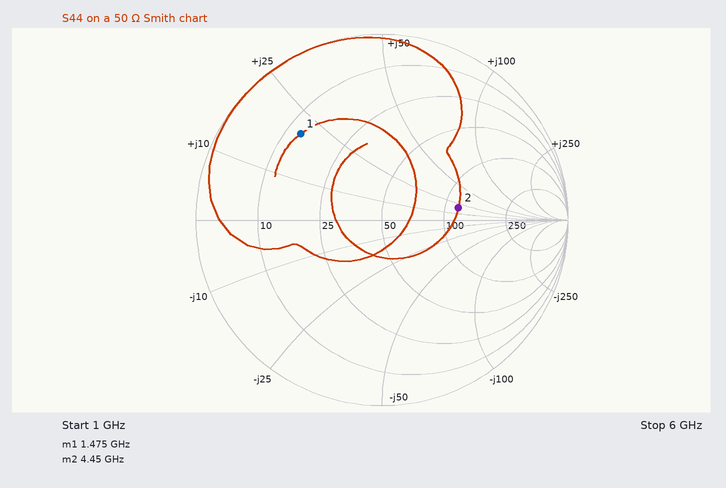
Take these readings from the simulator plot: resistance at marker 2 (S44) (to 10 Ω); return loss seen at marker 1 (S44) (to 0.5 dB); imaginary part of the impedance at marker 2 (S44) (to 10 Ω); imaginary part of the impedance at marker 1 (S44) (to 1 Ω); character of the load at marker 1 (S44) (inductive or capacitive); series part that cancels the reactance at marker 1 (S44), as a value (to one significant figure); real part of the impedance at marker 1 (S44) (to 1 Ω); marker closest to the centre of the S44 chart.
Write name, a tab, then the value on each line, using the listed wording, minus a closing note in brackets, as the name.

resistance at marker 2 (S44)	120 Ω
return loss seen at marker 1 (S44)	4.0 dB
imaginary part of the impedance at marker 2 (S44)	+20 Ω
imaginary part of the impedance at marker 1 (S44)	+20 Ω
character of the load at marker 1 (S44)	inductive
series part that cancels the reactance at marker 1 (S44), as a value	5 pF
real part of the impedance at marker 1 (S44)	13 Ω
marker closest to the centre of the S44 chart	marker 2
